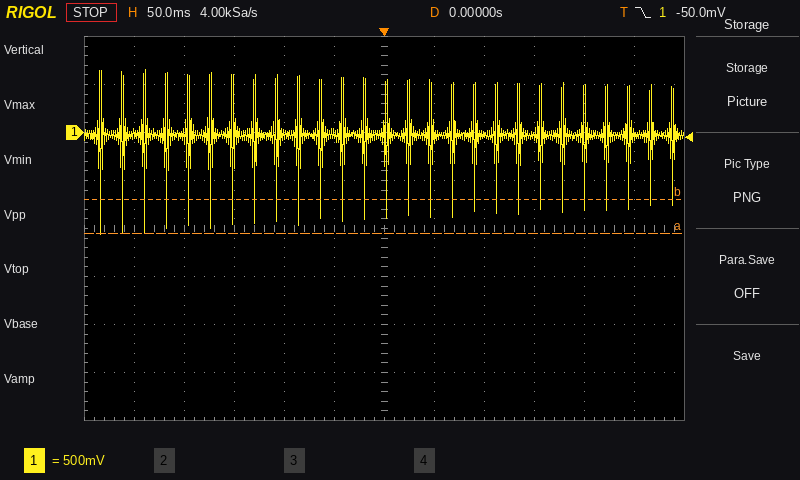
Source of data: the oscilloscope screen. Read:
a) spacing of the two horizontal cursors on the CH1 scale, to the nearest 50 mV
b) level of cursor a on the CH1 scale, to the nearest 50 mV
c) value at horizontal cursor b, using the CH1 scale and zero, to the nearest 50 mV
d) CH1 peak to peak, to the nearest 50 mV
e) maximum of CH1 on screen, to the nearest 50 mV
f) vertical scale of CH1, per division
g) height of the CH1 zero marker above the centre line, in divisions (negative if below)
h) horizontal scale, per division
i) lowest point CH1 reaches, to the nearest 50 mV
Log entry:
350 mV
-1.05 V
-700 mV
1.70 V
650 mV
500 mV
+2.0 div
50 ms
-1.05 V
